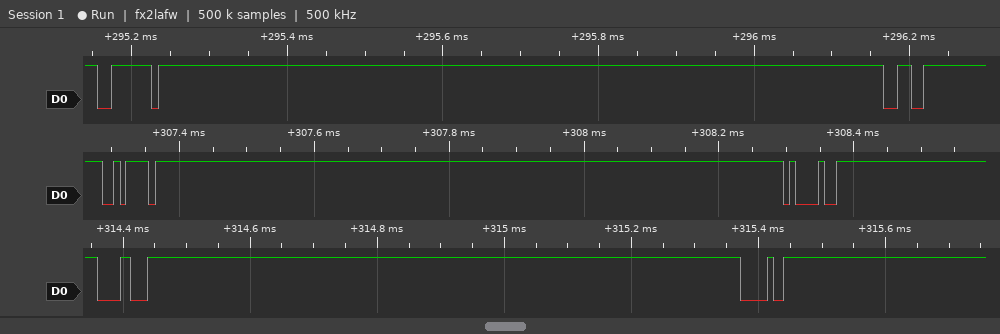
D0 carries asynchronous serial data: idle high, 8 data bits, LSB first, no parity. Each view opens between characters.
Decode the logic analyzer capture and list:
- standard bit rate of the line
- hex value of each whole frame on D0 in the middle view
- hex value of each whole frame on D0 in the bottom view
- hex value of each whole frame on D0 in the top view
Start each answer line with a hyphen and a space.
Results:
- 115200 baud
- 7A, 21
- 18, 90
- 7E, E6
